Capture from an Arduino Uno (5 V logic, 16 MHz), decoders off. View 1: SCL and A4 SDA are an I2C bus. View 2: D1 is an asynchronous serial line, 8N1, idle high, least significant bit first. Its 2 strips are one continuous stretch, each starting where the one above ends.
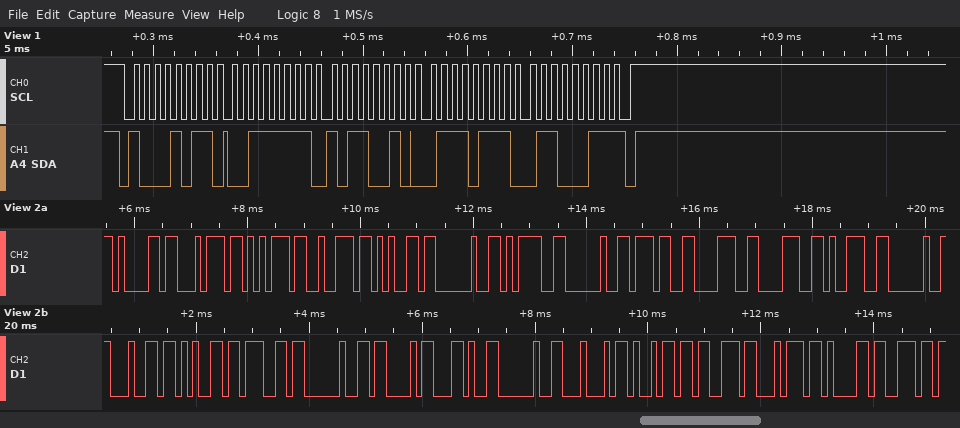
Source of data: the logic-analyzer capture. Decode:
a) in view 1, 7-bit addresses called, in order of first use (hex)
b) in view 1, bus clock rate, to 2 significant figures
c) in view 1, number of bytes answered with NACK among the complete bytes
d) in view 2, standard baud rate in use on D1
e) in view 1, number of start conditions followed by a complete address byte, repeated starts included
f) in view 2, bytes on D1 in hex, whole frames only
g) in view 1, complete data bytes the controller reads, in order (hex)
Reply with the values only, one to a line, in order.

0x45
100 kHz
1
9600 baud
1
61 74 75 72 65 20 3D 20 37 38 38 39 20 64 65 67 20 43 2C 20 44 69 73 74 61 6E
3F B2 77 63
